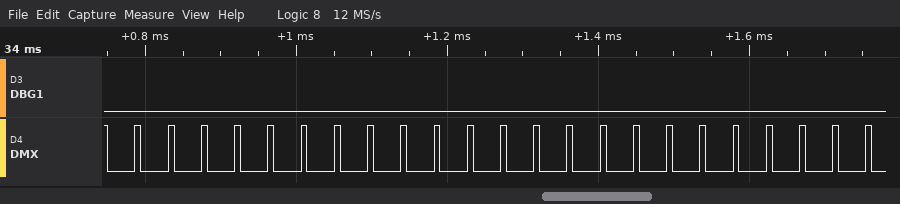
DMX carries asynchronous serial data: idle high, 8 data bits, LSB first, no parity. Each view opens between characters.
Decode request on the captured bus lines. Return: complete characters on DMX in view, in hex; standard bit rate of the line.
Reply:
08, 08, 08, 08, 08, 08, 08, 08, 08, 08, 08
115200 baud
